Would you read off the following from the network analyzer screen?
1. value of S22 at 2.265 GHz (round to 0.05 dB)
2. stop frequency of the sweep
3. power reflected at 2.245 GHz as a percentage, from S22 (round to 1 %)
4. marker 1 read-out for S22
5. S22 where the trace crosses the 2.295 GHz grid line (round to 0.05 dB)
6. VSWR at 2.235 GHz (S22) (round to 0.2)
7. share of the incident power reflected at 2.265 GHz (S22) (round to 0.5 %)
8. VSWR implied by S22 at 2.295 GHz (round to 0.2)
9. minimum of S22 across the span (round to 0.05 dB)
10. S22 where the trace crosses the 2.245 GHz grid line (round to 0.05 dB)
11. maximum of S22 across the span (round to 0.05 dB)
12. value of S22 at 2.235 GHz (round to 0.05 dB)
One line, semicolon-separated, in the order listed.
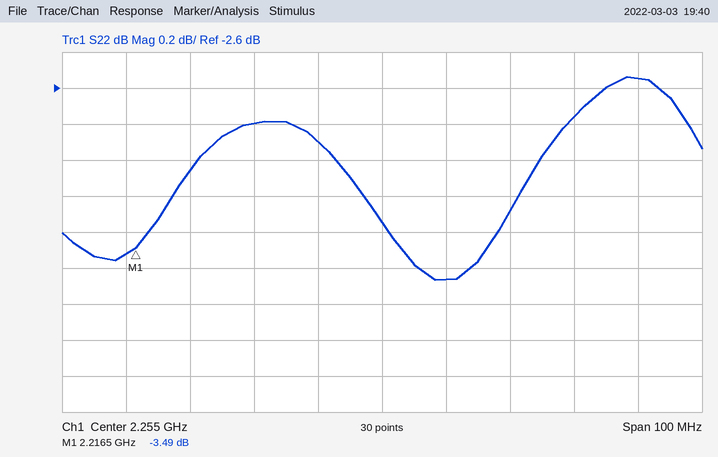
-3.65 dB; 2.305 GHz; 51 %; -3.49 dB; -2.55 dB; 6.2; 43.0 %; 6.8; -3.65 dB; -2.90 dB; -2.55 dB; -2.80 dB
